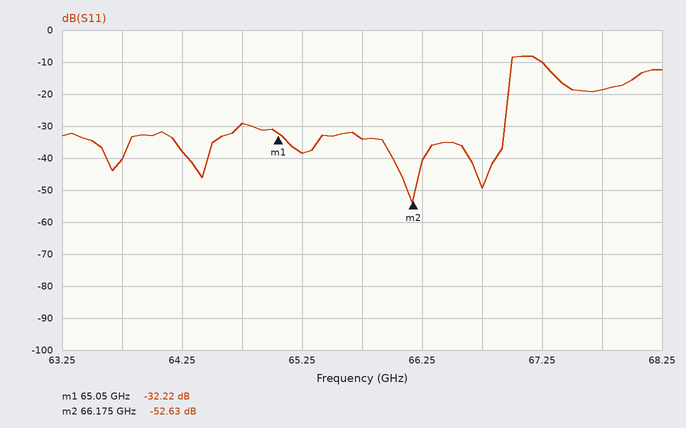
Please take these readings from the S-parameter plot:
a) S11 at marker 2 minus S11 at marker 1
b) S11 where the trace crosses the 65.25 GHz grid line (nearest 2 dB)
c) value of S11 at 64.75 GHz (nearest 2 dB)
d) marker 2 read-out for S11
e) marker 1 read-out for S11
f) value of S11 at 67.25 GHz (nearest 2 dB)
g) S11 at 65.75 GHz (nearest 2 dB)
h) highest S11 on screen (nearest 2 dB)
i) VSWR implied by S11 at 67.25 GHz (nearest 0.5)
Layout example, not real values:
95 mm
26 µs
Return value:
-20.41 dB
-38 dB
-30 dB
-52.63 dB
-32.22 dB
-10 dB
-34 dB
-8 dB
2.0
